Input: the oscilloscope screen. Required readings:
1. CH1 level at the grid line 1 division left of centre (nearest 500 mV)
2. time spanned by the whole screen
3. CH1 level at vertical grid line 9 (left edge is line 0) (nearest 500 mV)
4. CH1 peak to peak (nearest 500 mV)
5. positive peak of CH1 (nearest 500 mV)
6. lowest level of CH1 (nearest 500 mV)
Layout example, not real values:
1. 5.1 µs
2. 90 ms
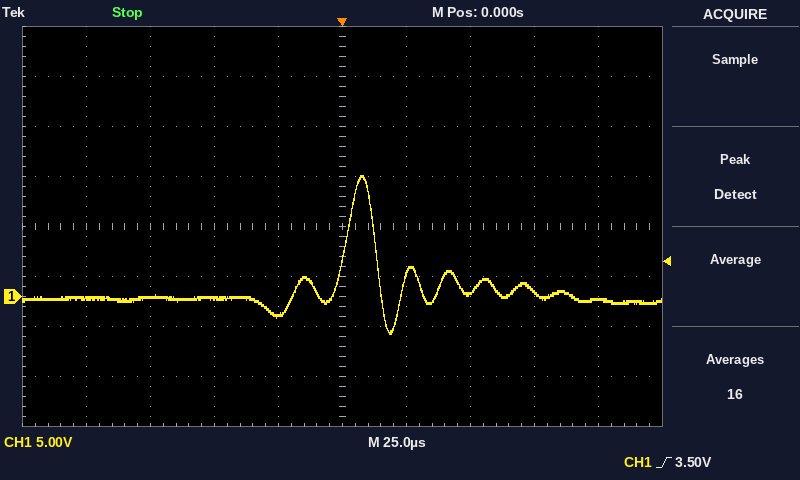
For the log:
1. -2.0 V
2. 250 µs
3. -500 mV
4. 16.0 V
5. 12.0 V
6. -4.0 V
